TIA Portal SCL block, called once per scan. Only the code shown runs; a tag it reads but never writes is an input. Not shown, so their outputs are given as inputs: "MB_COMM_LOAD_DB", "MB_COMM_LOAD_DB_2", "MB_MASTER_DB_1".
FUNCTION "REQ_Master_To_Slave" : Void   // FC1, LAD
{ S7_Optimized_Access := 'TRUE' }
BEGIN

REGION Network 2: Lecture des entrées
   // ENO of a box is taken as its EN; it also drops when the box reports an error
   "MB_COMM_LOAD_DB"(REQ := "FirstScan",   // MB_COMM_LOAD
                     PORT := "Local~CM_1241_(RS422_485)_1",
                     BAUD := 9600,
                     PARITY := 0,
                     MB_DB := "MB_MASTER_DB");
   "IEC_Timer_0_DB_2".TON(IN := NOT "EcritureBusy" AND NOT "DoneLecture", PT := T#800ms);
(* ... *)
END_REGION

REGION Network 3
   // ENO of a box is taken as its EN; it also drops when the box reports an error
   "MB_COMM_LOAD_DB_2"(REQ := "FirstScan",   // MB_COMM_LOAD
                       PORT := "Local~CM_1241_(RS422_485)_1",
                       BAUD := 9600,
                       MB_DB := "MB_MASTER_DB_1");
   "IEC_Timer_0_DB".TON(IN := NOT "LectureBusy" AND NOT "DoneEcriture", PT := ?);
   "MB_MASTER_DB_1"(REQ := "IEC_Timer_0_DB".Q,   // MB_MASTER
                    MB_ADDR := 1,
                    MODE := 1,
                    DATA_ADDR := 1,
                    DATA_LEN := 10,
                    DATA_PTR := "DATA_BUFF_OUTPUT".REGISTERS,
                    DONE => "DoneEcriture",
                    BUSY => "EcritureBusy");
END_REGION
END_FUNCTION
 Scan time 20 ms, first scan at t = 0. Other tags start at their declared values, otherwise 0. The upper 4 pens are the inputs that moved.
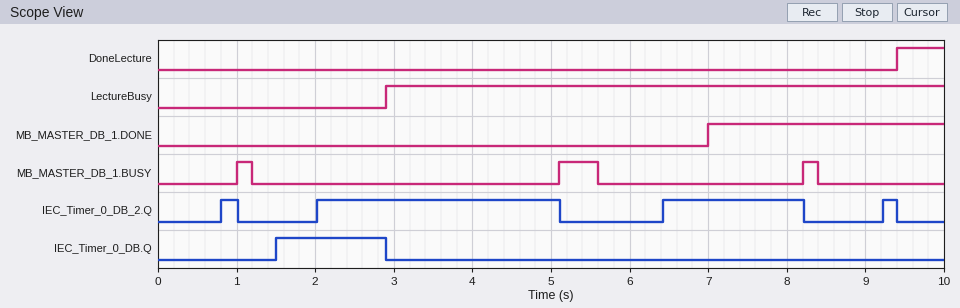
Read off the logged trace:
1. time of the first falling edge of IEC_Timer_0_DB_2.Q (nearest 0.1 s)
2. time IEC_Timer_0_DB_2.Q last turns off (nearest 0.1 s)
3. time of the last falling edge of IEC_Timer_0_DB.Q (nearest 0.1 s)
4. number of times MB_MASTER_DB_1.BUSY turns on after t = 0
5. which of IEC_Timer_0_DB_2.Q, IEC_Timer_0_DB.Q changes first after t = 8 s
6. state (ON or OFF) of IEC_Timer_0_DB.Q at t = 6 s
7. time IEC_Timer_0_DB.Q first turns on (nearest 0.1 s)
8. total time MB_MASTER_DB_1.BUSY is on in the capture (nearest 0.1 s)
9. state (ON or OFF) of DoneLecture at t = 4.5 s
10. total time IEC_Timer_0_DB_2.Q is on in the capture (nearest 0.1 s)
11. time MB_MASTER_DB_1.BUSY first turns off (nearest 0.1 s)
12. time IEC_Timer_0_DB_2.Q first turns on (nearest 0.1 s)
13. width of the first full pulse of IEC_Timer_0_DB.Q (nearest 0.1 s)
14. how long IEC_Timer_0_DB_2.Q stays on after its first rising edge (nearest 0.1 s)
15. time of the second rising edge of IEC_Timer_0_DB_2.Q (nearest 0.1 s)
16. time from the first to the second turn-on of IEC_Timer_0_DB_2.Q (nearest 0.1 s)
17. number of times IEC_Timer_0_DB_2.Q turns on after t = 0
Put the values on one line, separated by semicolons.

1.0 s; 9.4 s; 2.9 s; 3; IEC_Timer_0_DB_2.Q; OFF; 1.5 s; 0.9 s; OFF; 5.3 s; 1.2 s; 0.8 s; 1.4 s; 0.2 s; 2.0 s; 1.2 s; 4
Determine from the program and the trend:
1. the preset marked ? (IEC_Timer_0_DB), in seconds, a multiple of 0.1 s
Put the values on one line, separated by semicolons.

1.5 s
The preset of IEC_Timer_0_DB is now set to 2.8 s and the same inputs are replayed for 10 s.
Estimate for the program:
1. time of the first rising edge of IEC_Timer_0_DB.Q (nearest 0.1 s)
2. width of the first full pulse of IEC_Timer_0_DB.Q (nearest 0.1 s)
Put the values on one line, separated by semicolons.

2.8 s; 0.1 s
